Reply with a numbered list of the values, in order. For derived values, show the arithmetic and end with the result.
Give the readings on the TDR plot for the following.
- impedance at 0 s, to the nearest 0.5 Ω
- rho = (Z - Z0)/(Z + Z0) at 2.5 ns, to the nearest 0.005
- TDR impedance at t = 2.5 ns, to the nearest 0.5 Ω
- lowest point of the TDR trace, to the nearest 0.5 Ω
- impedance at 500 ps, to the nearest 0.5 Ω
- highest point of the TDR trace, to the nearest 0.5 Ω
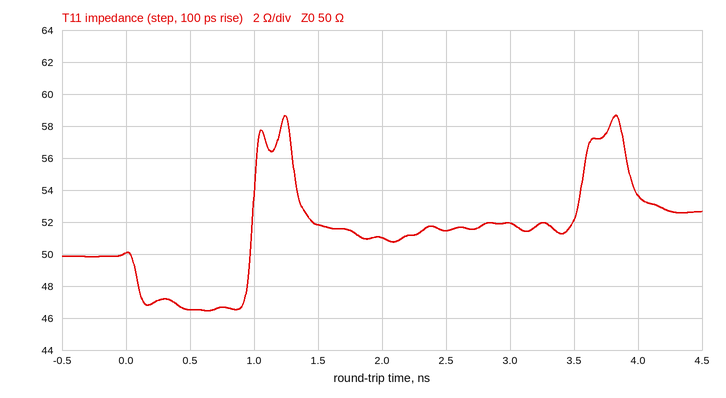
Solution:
1. 50.0 Ω
2. (51.5 − 50)/(51.5 + 50) ≈ +0.015
3. 51.5 Ω
4. 46.5 Ω
5. 46.5 Ω
6. 58.5 Ω
